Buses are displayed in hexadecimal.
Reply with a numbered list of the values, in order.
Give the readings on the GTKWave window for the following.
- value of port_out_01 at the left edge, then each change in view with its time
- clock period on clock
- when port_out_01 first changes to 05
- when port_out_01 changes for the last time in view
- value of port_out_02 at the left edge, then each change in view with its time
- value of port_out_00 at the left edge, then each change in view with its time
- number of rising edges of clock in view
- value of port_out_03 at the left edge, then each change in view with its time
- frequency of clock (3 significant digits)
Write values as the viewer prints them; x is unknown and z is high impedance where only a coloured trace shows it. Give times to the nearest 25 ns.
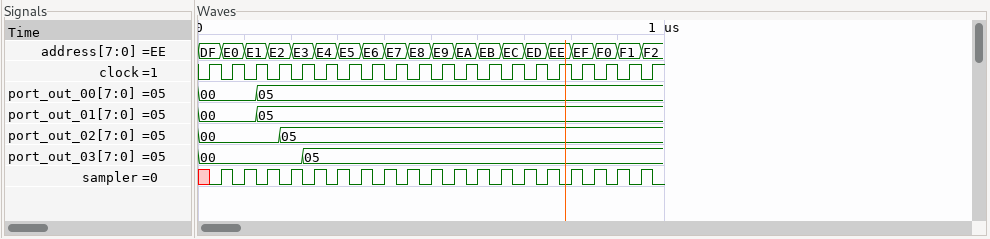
1. 00, 05 at 125 ns
2. 50 ns
3. 125 ns
4. 125 ns
5. 00, 05 at 175 ns
6. 00, 05 at 125 ns
7. 20
8. 00, 05 at 225 ns
9. 20.0 MHz
